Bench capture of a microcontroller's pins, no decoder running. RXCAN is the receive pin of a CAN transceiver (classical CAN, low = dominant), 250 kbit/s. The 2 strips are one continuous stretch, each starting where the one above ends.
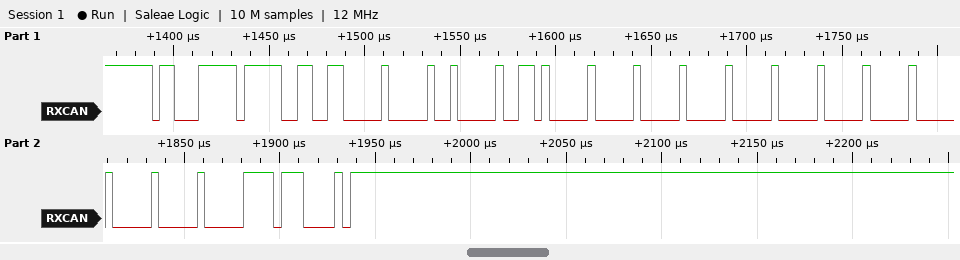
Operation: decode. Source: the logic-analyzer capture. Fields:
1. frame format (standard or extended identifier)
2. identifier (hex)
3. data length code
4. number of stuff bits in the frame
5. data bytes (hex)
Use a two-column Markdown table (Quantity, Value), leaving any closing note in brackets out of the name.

| Quantity | Value |
|---|---|
| frame format | extended |
| identifier | 0x18FF6600 |
| data length code | 8 |
| number of stuff bits in the frame | 17 |
| data bytes | 0D 00 00 00 00 00 00 00 |
